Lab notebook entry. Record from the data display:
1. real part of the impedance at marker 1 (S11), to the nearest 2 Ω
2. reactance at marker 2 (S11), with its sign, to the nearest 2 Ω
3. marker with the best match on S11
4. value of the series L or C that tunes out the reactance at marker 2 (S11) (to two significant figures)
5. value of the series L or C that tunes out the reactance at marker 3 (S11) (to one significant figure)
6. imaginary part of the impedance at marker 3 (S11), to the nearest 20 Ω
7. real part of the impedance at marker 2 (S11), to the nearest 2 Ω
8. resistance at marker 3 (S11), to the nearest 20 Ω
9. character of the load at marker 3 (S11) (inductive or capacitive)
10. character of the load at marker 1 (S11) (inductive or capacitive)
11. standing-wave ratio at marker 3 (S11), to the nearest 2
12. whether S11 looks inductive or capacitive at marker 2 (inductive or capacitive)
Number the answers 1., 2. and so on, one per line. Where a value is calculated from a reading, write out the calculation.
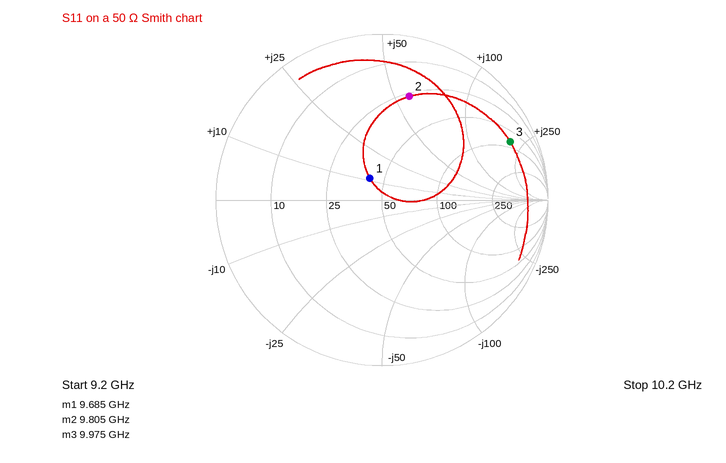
1. 42 Ω
2. +58 Ω
3. marker 1
4. C = 1/(2π × 9.805 GHz × 58 Ω) ≈ 280 fF
5. C = 1/(2π × 9.975 GHz × 200 Ω) ≈ 80 fF
6. +200 Ω
7. 26 Ω
8. 80 Ω
9. inductive
10. inductive
11. 12
12. inductive
